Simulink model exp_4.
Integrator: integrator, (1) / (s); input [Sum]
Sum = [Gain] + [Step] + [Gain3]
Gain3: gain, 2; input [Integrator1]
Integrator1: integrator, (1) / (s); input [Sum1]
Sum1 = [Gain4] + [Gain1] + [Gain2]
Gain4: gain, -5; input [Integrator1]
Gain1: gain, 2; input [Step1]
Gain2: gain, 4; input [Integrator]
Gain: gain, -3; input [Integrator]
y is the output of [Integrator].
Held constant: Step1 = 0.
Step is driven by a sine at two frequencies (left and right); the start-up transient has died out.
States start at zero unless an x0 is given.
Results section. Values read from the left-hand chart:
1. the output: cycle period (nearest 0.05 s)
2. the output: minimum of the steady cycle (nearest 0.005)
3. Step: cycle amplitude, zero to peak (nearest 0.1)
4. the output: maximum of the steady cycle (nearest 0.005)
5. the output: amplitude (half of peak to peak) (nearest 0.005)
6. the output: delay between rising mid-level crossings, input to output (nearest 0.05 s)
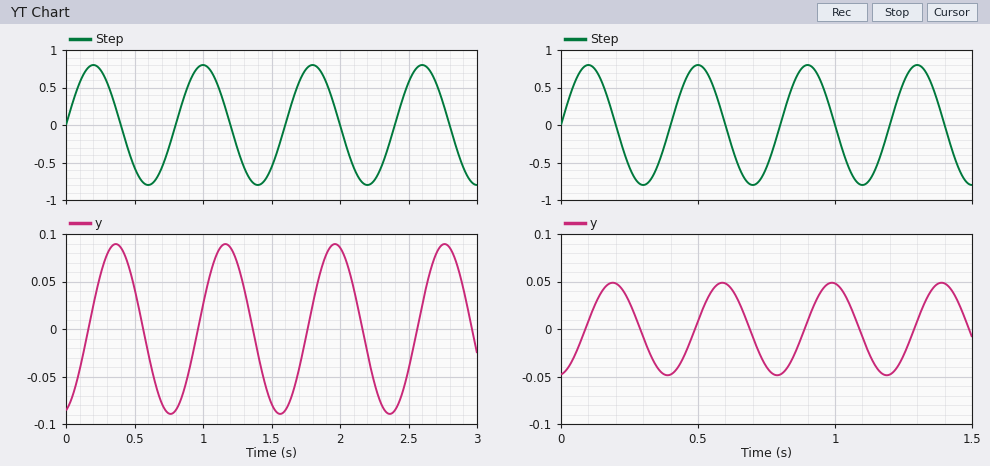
0.80 s
-0.090
0.8
0.090
0.090
0.15 s
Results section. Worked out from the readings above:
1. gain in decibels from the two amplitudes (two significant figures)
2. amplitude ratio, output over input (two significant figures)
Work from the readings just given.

-19 dB
0.11
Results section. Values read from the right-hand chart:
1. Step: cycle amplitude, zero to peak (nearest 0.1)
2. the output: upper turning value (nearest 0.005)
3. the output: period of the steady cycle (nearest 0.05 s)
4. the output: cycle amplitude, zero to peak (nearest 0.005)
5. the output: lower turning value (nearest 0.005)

0.8
0.050
0.40 s
0.050
-0.050
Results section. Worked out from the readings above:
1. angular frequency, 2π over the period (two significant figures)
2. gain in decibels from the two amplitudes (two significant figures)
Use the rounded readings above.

16 rad/s
-24 dB
